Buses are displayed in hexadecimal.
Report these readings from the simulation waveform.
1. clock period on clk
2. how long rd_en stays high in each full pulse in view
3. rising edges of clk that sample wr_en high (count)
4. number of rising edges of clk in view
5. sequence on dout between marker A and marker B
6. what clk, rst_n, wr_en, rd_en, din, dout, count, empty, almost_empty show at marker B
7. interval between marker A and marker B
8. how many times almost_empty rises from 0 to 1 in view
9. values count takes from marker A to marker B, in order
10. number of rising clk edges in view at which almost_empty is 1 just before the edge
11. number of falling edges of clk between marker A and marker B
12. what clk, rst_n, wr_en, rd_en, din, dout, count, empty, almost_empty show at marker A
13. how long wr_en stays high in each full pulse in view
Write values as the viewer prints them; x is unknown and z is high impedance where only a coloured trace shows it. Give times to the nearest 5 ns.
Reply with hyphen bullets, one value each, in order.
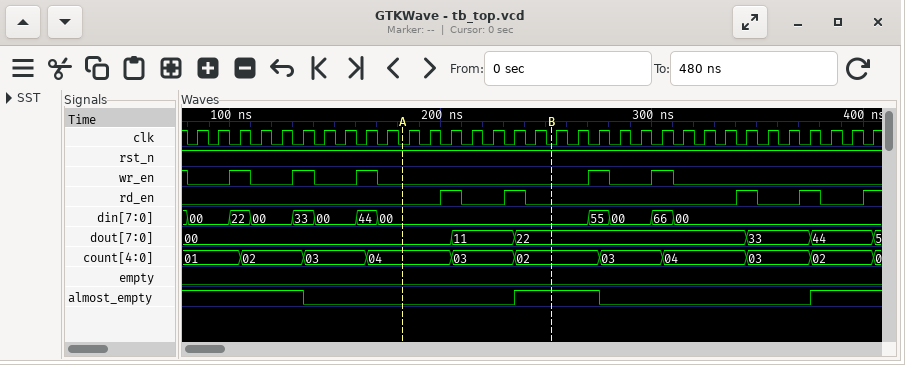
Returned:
- 10 ns
- 10 ns, 10 ns, 10 ns, 10 ns
- 5
- 33
- 00, 11, 22
- clk=0, rst_n=1, wr_en=0, rd_en=0, din=00, dout=22, count=02, empty=0, almost_empty=1
- 70 ns
- 2
- 04, 03, 02
- 13
- 7
- clk=0, rst_n=1, wr_en=0, rd_en=0, din=00, dout=00, count=04, empty=0, almost_empty=0
- 10 ns, 10 ns, 10 ns, 10 ns, 10 ns
